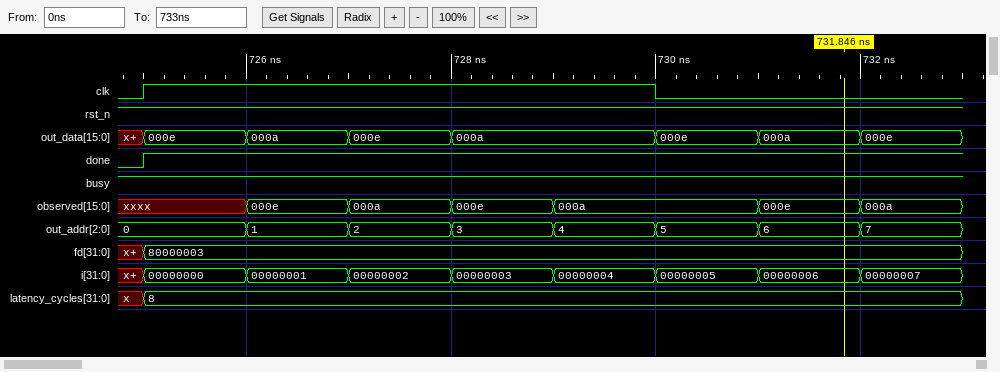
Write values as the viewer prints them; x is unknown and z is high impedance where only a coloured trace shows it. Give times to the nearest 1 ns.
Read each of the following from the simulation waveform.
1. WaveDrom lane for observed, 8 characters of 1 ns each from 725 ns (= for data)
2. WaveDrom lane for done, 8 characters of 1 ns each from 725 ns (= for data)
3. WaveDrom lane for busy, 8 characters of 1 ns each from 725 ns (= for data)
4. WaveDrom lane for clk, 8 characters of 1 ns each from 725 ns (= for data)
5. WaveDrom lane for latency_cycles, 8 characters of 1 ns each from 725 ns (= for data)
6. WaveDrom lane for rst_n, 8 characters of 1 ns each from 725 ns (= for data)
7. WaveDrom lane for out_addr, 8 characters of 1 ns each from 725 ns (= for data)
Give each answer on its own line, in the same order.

{name: 'observed', wave: 'x====.==', data: '000e 000a 000e 000a 000e 000a'}
{name: 'done', wave: '1.......'}
{name: 'busy', wave: '1.......'}
{name: 'clk', wave: '1....0..'}
{name: 'latency_cycles', wave: '=.......', data: '8'}
{name: 'rst_n', wave: '1.......'}
{name: 'out_addr', wave: '========', data: '0 1 2 3 4 5 6 7'}
